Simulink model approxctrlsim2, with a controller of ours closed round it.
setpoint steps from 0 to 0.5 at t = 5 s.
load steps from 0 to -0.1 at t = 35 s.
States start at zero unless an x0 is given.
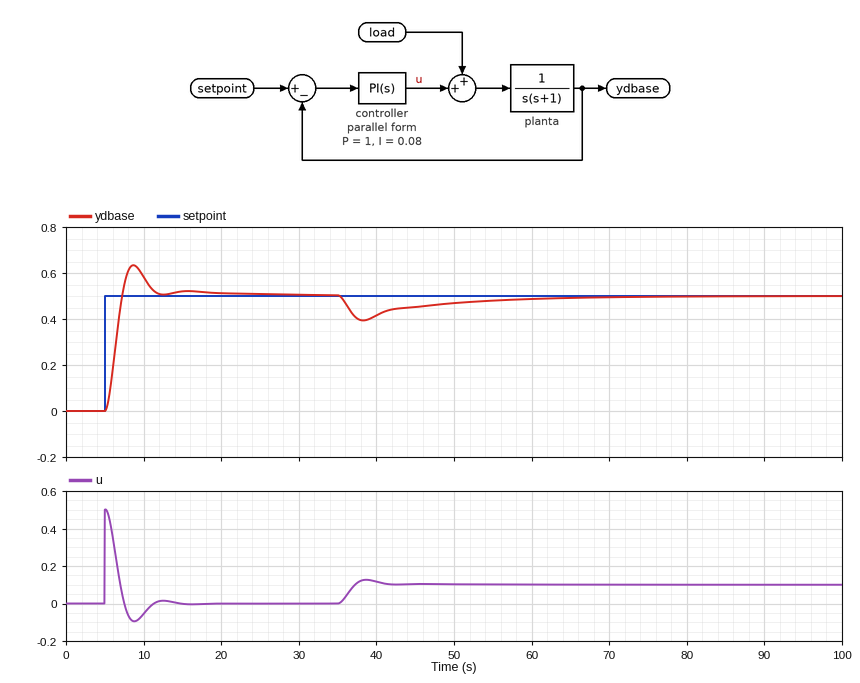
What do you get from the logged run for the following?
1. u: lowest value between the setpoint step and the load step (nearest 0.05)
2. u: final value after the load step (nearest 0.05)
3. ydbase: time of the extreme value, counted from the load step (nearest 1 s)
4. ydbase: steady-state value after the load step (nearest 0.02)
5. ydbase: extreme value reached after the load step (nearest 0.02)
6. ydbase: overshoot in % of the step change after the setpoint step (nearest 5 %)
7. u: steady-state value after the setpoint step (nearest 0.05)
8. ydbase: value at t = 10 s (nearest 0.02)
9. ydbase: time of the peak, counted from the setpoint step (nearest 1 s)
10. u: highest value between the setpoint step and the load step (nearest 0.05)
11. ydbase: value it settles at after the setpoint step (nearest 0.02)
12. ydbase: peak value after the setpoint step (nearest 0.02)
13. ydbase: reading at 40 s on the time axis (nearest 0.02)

-0.10
0.10
3 s
0.50
0.40
25 %
0.00
0.58
4 s
0.50
0.50
0.64
0.42
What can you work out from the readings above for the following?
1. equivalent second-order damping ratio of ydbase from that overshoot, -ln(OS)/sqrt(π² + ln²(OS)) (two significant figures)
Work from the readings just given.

0.40
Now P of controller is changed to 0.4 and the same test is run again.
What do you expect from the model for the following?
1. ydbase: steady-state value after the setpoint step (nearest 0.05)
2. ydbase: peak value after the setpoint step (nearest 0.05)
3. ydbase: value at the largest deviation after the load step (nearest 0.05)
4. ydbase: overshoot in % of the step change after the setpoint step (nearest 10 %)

0.50
0.70
0.30
40 %
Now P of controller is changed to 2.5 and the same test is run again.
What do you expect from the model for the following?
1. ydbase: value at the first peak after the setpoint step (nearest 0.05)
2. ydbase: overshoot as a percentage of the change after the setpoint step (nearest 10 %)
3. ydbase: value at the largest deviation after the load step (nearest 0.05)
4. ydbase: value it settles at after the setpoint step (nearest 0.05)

0.70
40 %
0.45
0.50
